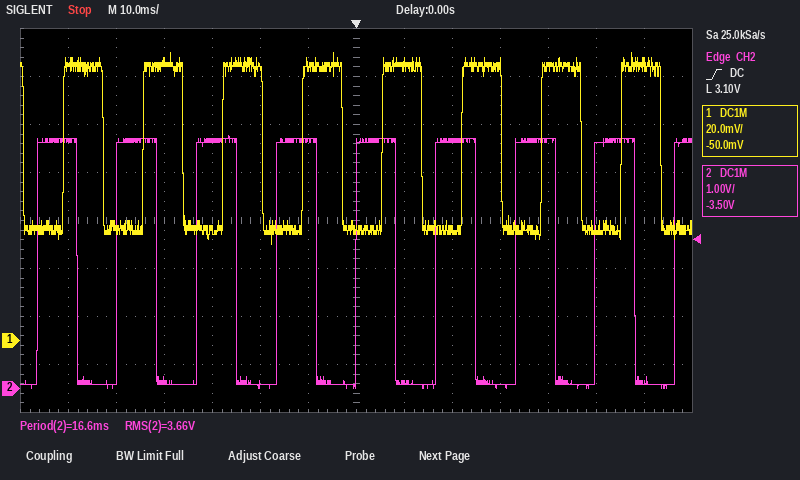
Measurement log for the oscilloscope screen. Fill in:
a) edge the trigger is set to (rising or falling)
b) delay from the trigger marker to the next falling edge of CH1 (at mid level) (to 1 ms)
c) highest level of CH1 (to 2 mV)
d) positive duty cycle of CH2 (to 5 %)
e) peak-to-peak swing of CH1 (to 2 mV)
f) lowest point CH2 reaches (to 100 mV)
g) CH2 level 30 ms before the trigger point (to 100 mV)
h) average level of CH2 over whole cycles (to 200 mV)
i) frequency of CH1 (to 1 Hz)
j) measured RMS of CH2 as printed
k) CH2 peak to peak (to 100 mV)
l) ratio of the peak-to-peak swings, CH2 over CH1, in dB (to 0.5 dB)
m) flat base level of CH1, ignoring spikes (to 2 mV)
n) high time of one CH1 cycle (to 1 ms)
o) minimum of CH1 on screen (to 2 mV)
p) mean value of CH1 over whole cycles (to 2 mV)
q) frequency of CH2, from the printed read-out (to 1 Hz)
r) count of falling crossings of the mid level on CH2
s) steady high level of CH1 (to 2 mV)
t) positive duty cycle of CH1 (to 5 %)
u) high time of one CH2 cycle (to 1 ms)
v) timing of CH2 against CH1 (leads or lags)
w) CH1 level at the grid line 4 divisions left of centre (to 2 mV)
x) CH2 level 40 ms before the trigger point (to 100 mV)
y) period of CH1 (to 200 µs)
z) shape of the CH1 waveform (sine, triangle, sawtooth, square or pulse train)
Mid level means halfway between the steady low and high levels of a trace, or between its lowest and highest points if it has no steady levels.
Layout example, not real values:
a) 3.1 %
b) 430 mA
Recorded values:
a) rising
b) 14 ms
c) 120 mV
d) 50 %
e) 80 mV
f) 0.0 V
g) 5.2 V
h) 2.6 V
i) 60 Hz
j) 3.66 V
k) 5.3 V
l) 36.5 dB
m) 46 mV
n) 8 ms
o) 40 mV
p) 80 mV
q) 60 Hz
r) 8
s) 114 mV
t) 50 %
u) 8 ms
v) leads
w) 116 mV
x) 200 mV
y) 16.6 ms
z) square
